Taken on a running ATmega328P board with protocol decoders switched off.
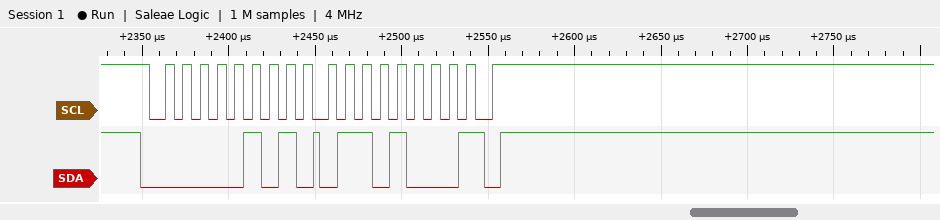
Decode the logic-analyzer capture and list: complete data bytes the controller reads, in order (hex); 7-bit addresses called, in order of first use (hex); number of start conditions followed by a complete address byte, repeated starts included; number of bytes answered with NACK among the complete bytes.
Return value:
68
0x02
1
1
